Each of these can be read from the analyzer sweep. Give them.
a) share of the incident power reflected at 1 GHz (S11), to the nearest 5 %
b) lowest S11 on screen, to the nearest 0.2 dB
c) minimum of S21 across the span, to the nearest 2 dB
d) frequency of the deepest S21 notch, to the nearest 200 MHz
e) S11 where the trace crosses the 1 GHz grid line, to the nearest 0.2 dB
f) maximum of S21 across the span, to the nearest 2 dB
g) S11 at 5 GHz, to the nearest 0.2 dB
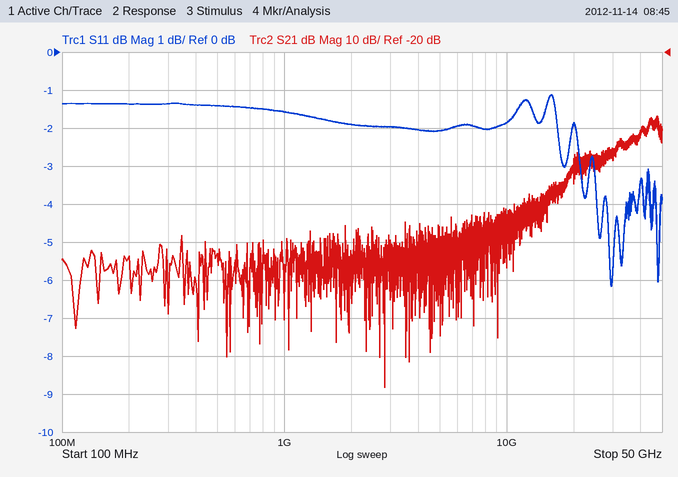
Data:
70 %
-6.2 dB
-108 dB
2.8 GHz
-1.6 dB
-36 dB
-2.0 dB
